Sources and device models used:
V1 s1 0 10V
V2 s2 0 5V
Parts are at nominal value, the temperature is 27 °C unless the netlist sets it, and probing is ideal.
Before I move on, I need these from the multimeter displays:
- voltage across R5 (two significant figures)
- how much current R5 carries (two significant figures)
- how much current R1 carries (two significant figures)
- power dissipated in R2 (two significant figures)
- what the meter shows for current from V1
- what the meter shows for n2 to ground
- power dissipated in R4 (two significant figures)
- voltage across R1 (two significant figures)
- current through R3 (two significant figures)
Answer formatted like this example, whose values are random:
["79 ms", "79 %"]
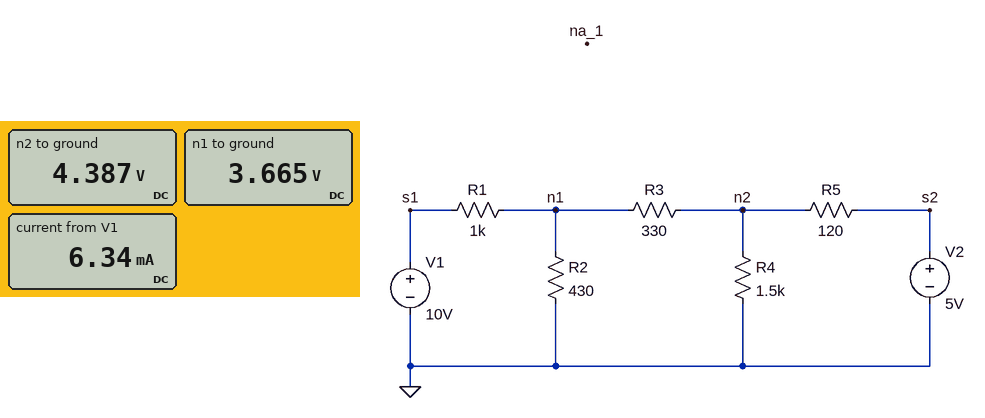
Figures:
["610 mV", "5.1 mA", "6.3 mA", "31 mW", "6.34 mA", "4.387 V", "13 mW", "6.3 V", "2.2 mA"]
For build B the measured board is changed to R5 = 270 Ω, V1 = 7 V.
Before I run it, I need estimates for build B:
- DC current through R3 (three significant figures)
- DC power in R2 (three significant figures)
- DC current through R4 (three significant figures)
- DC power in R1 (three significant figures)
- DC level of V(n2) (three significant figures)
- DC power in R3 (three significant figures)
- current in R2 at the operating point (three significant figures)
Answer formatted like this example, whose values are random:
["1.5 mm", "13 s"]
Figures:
["2.48 mA", "18.9 mW", "2.45 mA", "17.2 mW", "3.67 V", "2.03 mW", "6.63 mA"]
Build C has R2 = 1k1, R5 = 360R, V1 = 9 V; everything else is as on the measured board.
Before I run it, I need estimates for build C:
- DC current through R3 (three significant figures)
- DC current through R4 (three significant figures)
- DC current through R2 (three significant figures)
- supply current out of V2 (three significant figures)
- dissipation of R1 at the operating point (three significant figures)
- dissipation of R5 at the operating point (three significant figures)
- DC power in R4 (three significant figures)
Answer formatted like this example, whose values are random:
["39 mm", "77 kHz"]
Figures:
["596 µA", "2.80 mA", "4.00 mA", "2.21 mA", "21.1 mW", "1.75 mW", "11.8 mW"]
